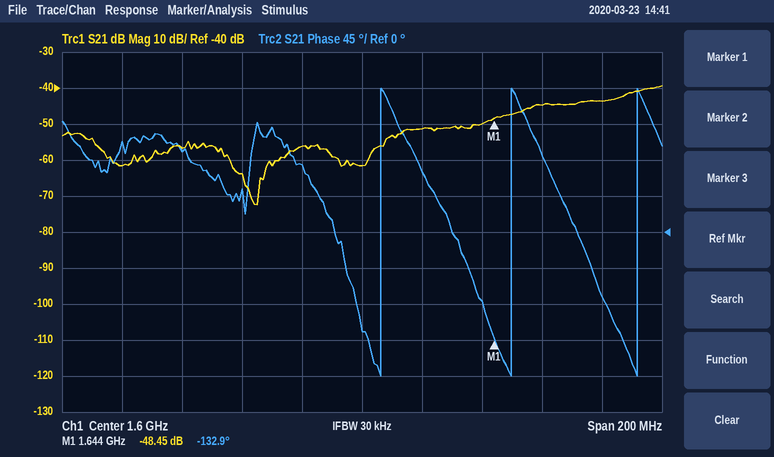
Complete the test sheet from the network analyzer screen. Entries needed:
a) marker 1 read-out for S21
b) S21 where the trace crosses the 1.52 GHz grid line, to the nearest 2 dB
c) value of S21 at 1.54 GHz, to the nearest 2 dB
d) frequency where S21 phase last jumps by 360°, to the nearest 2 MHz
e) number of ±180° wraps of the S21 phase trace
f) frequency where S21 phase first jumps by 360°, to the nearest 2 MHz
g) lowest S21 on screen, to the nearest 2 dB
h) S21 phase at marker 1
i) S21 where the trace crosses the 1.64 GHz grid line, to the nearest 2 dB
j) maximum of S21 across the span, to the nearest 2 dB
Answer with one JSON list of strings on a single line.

["-48.45 dB", "-62 dB", "-56 dB", "1.692 GHz", "3", "1.606 GHz", "-72 dB", "-132.9°", "-50 dB", "-40 dB"]
